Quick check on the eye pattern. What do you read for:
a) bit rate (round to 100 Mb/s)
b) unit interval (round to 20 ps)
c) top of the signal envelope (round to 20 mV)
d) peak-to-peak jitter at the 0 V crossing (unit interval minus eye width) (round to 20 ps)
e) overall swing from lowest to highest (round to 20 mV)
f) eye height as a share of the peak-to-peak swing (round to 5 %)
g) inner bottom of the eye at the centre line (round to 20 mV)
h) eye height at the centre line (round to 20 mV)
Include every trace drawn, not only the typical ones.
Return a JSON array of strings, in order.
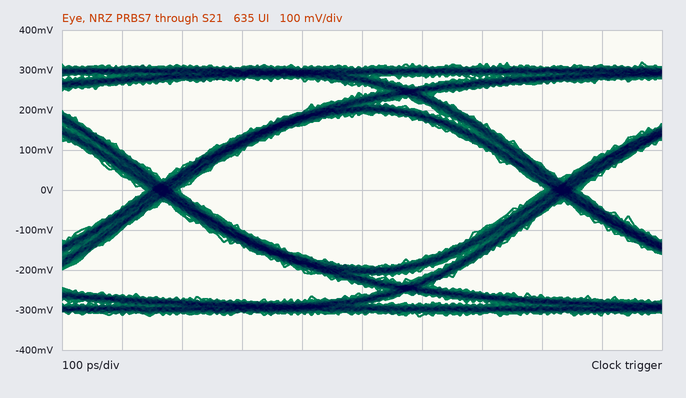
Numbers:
["1.5 Gb/s", "660 ps", "320 mV", "60 ps", "640 mV", "60 %", "-200 mV", "380 mV"]
